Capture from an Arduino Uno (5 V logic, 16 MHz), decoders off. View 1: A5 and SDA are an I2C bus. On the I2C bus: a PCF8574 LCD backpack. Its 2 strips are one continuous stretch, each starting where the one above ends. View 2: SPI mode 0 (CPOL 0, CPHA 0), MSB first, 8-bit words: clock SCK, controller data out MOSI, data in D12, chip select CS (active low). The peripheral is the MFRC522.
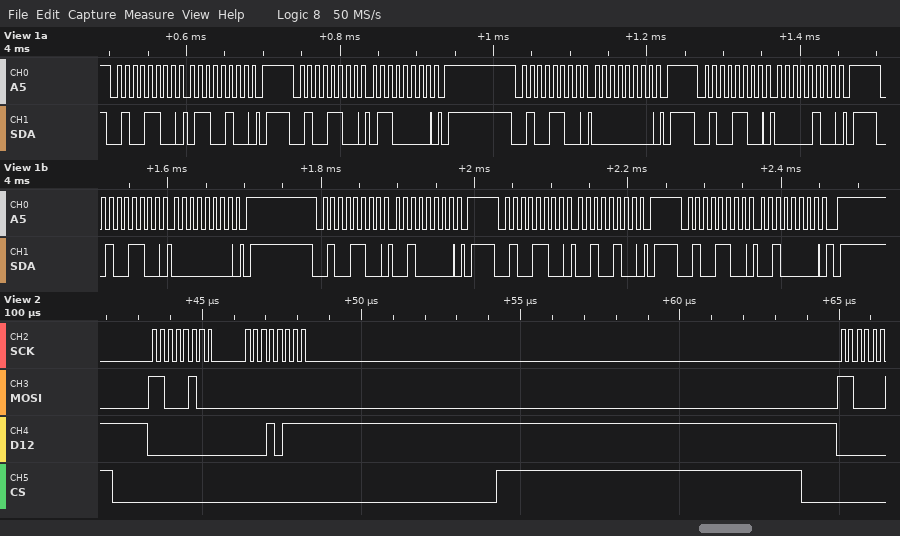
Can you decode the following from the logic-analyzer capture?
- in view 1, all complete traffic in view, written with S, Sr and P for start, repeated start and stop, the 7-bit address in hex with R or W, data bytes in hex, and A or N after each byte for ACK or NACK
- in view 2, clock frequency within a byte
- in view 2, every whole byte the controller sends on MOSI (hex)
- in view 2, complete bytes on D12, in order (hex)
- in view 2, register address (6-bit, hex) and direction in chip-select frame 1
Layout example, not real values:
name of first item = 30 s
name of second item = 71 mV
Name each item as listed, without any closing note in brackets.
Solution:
in view 1, all complete traffic in view, written with S, Sr and P for start, repeated start and stop, the 7-bit address in hex with R or W, data bytes in hex, and A or N after each byte for ACK or NACK = S 26W A 64 A P S 26W A 60 A P S 26W A 00 A P S 26W A 04 A P S 26W A 00 A P S 26W A 20 A P S 26W A 24 A P S 26W A 20 A P
in view 2, clock frequency within a byte = 4 MHz
in view 2, every whole byte the controller sends on MOSI = C4 00
in view 2, complete bytes on D12, in order = 00 17
in view 2, register address (6-bit, hex) and direction in chip-select frame 1 = 0x22 read
